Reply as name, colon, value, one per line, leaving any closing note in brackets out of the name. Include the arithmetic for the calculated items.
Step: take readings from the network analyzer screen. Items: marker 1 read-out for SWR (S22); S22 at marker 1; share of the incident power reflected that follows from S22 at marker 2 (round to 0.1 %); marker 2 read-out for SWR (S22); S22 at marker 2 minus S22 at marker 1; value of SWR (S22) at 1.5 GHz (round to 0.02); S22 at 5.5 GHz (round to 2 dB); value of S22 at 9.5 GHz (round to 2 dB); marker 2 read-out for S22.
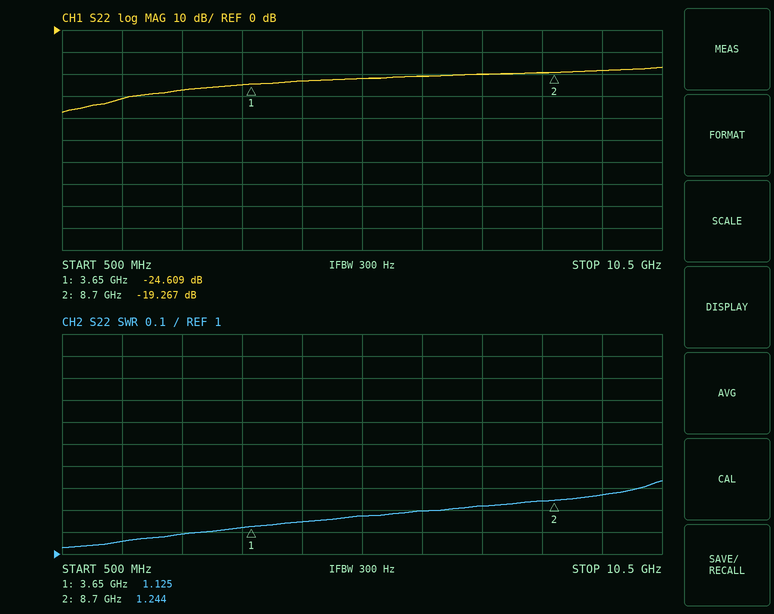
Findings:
marker 1 read-out for SWR: 1.125
S22 at marker 1: -24.609 dB
share of the incident power reflected that follows from S22 at marker 2: 10^(-19.267/10) ≈ 1.2 %
marker 2 read-out for SWR: 1.244
S22 at marker 2 minus S22 at marker 1: -19.267 − (-24.609) = 5.342 dB
value of SWR (S22) at 1.5 GHz: 1.06
S22 at 5.5 GHz: -22 dB
value of S22 at 9.5 GHz: -18 dB
marker 2 read-out for S22: -19.267 dB
